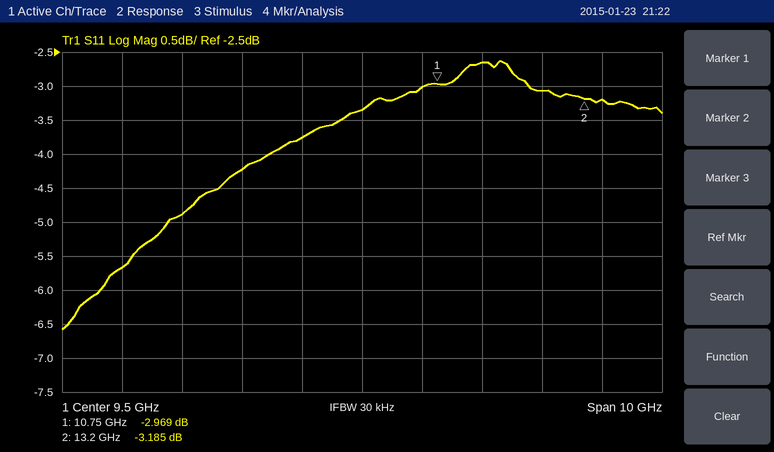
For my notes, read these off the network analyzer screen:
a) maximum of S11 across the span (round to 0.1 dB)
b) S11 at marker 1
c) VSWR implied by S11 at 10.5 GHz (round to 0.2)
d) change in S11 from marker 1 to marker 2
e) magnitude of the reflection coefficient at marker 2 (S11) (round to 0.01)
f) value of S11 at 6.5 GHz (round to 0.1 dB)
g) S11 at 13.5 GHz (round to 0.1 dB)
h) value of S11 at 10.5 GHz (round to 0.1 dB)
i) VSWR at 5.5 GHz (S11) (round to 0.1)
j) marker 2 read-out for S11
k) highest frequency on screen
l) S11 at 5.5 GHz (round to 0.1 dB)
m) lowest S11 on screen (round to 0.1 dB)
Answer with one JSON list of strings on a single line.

["-2.6 dB", "-2.969 dB", "5.8", "-0.216 dB", "0.69", "-4.9 dB", "-3.2 dB", "-3.0 dB", "3.2", "-3.185 dB", "14.5 GHz", "-5.7 dB", "-6.6 dB"]
